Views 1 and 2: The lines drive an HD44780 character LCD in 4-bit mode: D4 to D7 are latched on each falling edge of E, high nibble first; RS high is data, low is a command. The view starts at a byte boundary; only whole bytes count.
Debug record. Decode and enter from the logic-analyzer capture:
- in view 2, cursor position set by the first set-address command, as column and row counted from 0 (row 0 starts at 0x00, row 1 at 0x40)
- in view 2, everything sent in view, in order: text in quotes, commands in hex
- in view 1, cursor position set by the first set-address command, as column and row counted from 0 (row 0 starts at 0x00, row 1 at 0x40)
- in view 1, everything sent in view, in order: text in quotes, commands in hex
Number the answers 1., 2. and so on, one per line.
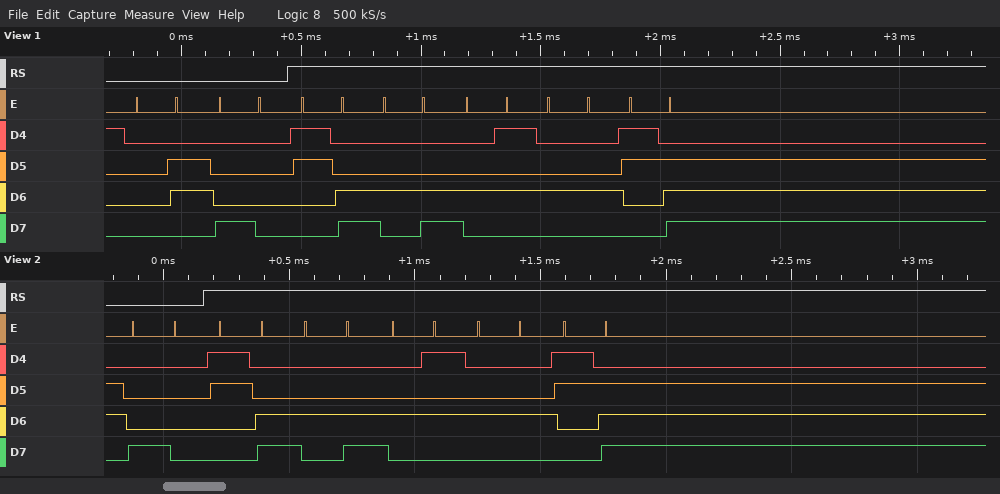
1. column 0, row 0
2. 0x80 "<LED>"
3. column 0, row 0
4. 0x06 0x80 "<LED>"
